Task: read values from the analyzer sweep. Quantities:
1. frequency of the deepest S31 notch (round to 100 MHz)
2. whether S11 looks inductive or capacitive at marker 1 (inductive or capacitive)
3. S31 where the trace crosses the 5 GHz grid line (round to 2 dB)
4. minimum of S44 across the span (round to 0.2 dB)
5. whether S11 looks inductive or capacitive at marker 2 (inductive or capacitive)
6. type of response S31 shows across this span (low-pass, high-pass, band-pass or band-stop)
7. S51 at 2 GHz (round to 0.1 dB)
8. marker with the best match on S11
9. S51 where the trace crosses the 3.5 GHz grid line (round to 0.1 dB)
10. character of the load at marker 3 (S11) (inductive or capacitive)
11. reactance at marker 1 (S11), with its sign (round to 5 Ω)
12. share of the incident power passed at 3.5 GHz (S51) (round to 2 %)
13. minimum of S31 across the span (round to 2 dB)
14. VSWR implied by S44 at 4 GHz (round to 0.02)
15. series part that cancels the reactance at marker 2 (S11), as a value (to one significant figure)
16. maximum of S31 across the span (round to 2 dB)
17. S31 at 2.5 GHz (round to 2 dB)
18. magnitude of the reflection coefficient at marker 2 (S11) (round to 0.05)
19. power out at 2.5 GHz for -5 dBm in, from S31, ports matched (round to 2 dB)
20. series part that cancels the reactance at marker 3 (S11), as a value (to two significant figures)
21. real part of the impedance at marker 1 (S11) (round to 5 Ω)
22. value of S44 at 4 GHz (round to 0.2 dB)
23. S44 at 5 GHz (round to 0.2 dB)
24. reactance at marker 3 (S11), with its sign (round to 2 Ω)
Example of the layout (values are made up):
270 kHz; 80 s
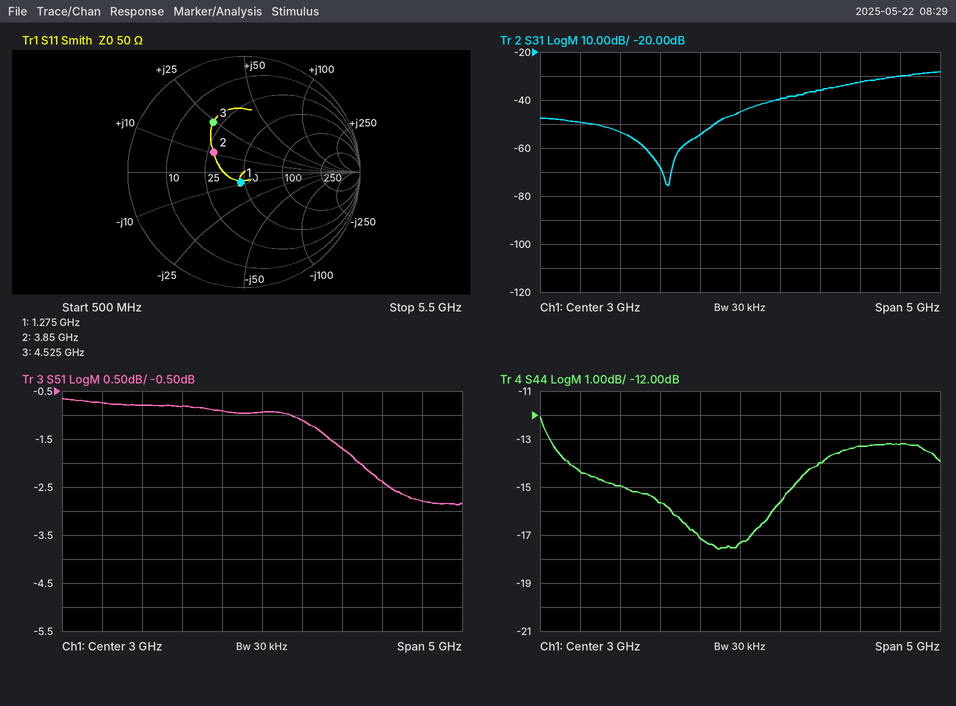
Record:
2.1 GHz; capacitive; -30 dB; -17.6 dB; inductive; high-pass; -0.8 dB; marker 1; -1.1 dB; inductive; -10 Ω; 78 %; -76 dB; 1.50; 4 pF; -28 dB; -54 dB; 0.30; -60 dBm; 1.5 pF; 45 Ω; -14.0 dB; -13.2 dB; +24 Ω
